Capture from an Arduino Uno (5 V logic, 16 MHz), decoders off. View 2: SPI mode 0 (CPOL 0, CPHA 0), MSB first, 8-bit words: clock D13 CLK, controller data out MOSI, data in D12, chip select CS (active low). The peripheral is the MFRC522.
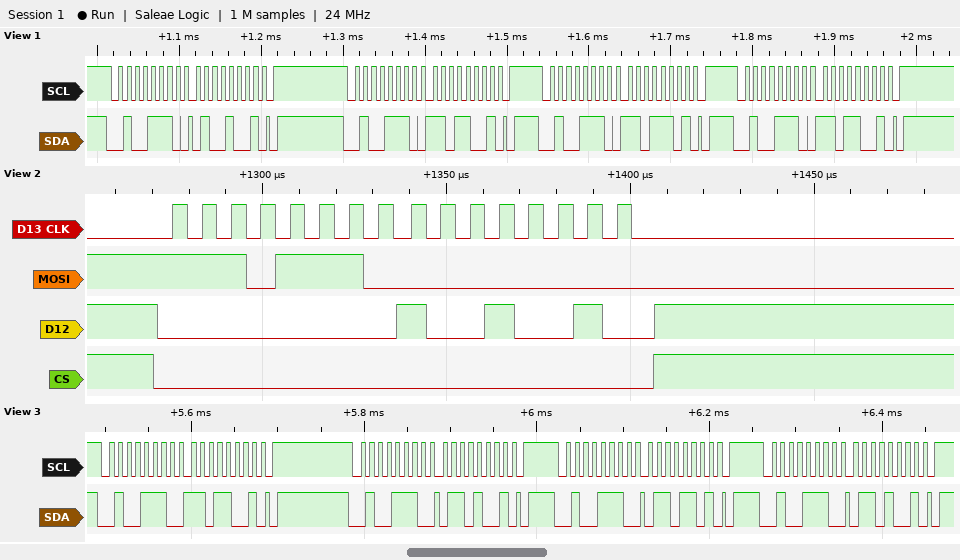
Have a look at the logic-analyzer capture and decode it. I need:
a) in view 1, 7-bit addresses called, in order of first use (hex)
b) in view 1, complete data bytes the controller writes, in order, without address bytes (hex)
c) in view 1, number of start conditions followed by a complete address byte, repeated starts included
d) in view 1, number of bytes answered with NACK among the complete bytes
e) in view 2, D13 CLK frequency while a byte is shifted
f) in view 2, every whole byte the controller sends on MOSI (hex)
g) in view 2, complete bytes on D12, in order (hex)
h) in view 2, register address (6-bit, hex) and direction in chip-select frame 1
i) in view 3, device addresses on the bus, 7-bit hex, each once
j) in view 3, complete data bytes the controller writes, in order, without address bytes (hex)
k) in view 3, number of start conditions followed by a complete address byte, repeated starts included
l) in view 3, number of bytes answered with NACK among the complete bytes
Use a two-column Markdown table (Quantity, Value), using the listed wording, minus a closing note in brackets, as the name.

| Quantity | Value |
|---|---|
| in view 1, 7-bit addresses called, in order of first use | 0x27 |
| in view 1, complete data bytes the controller writes, in order, without address bytes | 49 D9 DD D9 |
| in view 1, number of start conditions followed by a complete address byte, repeated starts included | 4 |
| in view 1, number of bytes answered with NACK among the complete bytes | 0 |
| in view 2, D13 CLK frequency while a byte is shifted | 125 kHz |
| in view 2, every whole byte the controller sends on MOSI | 0xEE 0x00 |
| in view 2, complete bytes on D12, in order | 0x00 0x92 |
| in view 2, register address (6-bit, hex) and direction in chip-select frame 1 | 0x37 read |
| in view 3, device addresses on the bus, 7-bit hex, each once | 0x27 |
| in view 3, complete data bytes the controller writes, in order, without address bytes | D9 69 6D 69 |
| in view 3, number of start conditions followed by a complete address byte, repeated starts included | 4 |
| in view 3, number of bytes answered with NACK among the complete bytes | 0 |
